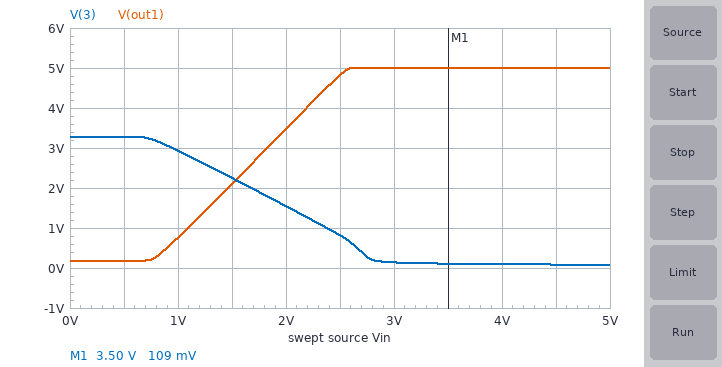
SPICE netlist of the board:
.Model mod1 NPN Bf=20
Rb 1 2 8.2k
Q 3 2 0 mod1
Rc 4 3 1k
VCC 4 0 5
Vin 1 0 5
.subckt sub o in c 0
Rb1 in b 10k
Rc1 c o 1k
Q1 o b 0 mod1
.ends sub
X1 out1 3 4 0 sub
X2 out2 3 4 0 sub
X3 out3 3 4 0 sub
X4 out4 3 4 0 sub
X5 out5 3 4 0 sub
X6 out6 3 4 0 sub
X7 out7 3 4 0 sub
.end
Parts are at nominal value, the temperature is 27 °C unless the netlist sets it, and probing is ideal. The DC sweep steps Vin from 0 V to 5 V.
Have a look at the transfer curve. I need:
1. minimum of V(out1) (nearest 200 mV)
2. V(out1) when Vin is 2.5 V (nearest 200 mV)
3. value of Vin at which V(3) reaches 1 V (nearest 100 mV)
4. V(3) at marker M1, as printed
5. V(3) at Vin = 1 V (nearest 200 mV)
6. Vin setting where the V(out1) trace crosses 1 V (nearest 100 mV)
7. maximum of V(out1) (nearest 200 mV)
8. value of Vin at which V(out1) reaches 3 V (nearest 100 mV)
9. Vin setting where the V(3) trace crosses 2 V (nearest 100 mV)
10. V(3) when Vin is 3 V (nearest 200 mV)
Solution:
200 mV
4.8 V
2.4 V
109 mV
3.0 V
1.1 V
5.0 V
1.8 V
1.7 V
200 mV
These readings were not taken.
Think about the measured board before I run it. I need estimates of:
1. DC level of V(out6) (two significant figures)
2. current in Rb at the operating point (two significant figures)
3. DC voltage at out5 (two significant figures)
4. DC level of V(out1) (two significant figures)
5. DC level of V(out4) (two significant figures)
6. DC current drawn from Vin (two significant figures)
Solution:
5.0 V
510 µA
5.0 V
5.0 V
5.0 V
510 µA
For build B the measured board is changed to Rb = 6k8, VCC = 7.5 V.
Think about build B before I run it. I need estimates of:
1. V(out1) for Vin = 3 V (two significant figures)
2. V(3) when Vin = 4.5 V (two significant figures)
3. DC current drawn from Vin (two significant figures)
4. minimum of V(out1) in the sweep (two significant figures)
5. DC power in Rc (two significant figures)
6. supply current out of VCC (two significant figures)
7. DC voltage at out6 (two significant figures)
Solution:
7.1 V
100 mV
610 µA
150 mV
55 mW
7.4 mA
7.5 V
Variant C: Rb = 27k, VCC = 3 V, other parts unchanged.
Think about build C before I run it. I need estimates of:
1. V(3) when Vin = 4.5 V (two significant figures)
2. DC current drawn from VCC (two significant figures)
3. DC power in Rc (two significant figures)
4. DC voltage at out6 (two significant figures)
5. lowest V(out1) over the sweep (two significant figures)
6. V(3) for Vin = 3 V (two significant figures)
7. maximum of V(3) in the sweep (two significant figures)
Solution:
260 mV
2.9 mA
8.2 mW
3.0 V
410 mV
1.1 V
2.1 V
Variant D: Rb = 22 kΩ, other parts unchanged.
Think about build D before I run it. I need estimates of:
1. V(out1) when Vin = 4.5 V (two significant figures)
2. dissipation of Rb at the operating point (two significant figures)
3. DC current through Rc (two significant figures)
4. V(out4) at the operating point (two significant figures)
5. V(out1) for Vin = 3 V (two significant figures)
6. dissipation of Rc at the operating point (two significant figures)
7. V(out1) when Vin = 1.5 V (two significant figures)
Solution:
4.0 V
800 µW
4.0 mA
4.5 V
2.4 V
16 mW
860 mV
